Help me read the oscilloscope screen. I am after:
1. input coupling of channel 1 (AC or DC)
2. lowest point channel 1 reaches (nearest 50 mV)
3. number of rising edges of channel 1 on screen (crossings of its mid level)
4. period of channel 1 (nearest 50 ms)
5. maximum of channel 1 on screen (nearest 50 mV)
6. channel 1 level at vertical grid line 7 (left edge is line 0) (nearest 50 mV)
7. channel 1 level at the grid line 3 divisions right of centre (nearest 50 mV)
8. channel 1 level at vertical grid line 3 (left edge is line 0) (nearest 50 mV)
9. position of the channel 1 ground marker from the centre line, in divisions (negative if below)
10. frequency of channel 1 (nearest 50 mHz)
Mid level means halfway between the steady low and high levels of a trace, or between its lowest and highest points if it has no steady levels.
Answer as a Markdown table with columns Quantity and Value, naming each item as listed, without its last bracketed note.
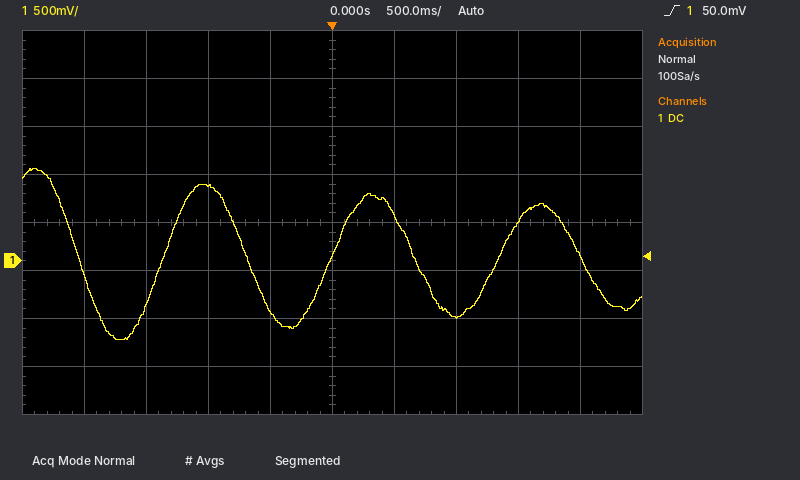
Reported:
| Quantity | Value |
|---|---|
| input coupling of channel 1 | DC |
| lowest point channel 1 reaches | -800 mV |
| number of rising edges of channel 1 on screen | 3 |
| period of channel 1 | 1.35 s |
| maximum of channel 1 on screen | 950 mV |
| channel 1 level at vertical grid line 7 (left edge is line 0) | -600 mV |
| channel 1 level at the grid line 3 divisions right of centre | 400 mV |
| channel 1 level at vertical grid line 3 (left edge is line 0) | 800 mV |
| position of the channel 1 ground marker from the centre line, in divisions | -0.8 div |
| frequency of channel 1 | 750 mHz |
